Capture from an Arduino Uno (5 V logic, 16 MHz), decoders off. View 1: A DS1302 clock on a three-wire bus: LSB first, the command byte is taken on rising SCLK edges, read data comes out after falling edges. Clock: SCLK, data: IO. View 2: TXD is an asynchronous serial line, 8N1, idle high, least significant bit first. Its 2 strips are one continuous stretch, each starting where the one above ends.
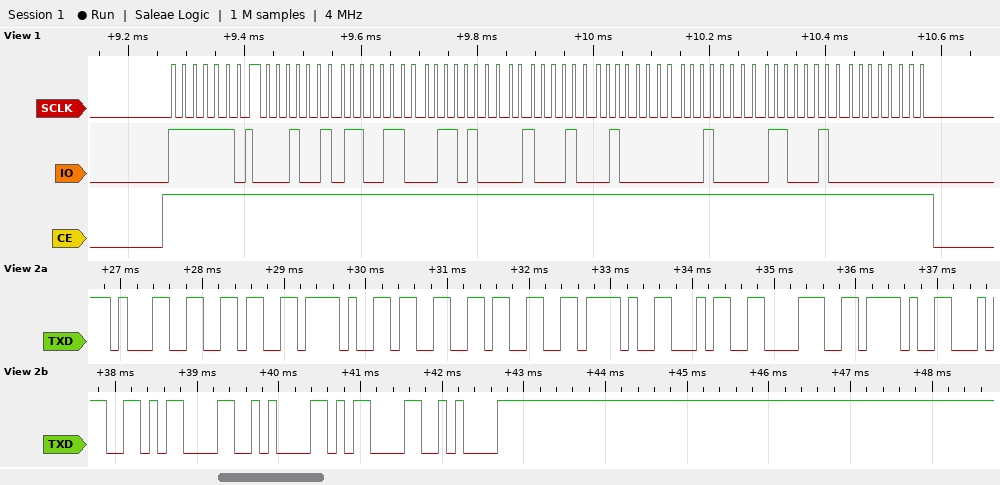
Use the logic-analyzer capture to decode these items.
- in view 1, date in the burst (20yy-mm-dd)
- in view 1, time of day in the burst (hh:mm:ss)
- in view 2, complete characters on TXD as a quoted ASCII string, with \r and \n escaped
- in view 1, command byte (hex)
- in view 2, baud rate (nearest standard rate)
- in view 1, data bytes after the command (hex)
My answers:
2023-02-22
16:33:48
"16/33/48/4\r\n\r\n"
0xBF
9600 baud
48 33 16 22 02 04 23 00
